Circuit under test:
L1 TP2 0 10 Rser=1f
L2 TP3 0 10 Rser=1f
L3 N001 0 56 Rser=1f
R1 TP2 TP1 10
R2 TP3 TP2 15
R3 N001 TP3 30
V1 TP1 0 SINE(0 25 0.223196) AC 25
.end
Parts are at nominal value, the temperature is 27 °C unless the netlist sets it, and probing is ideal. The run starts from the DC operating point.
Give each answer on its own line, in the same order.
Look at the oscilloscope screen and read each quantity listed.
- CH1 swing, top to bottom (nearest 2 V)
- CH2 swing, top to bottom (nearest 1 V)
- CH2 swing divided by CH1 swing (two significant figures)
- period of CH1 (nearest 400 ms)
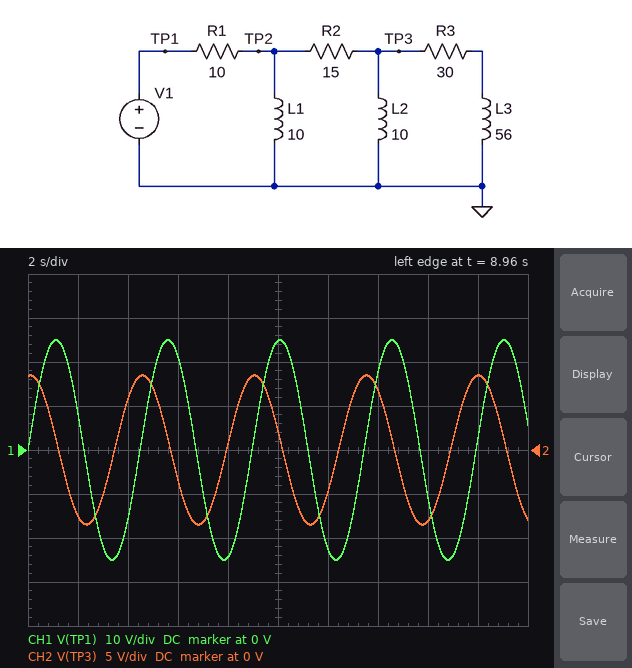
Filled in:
50 V
17 V
0.34
4.4 s
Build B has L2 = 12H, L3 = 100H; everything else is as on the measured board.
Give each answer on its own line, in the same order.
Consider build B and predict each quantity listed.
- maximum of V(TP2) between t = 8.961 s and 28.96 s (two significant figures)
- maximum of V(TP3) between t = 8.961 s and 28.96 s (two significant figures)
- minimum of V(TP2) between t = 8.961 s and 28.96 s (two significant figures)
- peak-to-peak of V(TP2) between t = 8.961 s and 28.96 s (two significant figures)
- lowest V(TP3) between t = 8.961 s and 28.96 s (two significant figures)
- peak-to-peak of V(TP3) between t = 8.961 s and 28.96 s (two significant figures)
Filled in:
15 V
10 V
-15 V
29 V
-10 V
20 V
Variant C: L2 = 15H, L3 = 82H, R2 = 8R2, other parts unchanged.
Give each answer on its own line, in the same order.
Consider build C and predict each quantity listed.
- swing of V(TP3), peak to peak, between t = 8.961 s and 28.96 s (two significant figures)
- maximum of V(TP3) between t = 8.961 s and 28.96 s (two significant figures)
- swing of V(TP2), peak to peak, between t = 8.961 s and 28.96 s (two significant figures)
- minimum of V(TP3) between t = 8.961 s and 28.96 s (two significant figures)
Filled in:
26 V
13 V
29 V
-13 V
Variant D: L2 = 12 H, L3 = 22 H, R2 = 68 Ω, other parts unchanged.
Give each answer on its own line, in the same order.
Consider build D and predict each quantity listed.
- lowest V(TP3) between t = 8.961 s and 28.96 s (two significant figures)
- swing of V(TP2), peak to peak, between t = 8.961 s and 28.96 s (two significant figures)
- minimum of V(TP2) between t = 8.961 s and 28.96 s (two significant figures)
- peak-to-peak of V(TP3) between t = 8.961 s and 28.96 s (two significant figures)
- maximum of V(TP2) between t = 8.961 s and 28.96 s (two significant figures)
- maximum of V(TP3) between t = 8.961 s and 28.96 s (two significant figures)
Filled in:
-3.2 V
36 V
-18 V
6.4 V
18 V
3.2 V
